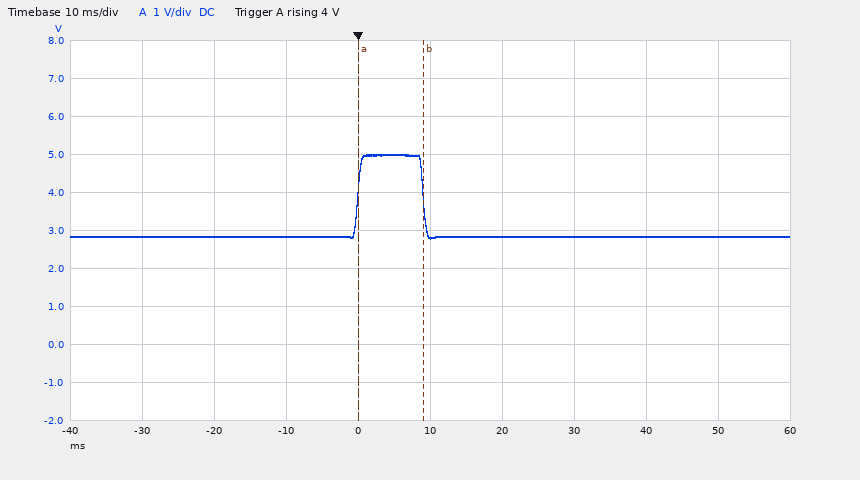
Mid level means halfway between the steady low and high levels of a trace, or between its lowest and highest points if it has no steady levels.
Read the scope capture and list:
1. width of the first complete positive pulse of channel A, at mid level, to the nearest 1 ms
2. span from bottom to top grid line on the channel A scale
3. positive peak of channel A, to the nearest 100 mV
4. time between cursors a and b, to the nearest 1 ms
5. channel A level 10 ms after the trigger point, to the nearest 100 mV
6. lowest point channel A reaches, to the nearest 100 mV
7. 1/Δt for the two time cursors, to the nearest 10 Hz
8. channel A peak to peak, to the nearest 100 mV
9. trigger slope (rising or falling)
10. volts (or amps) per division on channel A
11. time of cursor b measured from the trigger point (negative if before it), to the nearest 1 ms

9 ms
10 V
5.0 V
9 ms
2.9 V
2.8 V
110 Hz
2.2 V
rising
1 V
+9 ms
